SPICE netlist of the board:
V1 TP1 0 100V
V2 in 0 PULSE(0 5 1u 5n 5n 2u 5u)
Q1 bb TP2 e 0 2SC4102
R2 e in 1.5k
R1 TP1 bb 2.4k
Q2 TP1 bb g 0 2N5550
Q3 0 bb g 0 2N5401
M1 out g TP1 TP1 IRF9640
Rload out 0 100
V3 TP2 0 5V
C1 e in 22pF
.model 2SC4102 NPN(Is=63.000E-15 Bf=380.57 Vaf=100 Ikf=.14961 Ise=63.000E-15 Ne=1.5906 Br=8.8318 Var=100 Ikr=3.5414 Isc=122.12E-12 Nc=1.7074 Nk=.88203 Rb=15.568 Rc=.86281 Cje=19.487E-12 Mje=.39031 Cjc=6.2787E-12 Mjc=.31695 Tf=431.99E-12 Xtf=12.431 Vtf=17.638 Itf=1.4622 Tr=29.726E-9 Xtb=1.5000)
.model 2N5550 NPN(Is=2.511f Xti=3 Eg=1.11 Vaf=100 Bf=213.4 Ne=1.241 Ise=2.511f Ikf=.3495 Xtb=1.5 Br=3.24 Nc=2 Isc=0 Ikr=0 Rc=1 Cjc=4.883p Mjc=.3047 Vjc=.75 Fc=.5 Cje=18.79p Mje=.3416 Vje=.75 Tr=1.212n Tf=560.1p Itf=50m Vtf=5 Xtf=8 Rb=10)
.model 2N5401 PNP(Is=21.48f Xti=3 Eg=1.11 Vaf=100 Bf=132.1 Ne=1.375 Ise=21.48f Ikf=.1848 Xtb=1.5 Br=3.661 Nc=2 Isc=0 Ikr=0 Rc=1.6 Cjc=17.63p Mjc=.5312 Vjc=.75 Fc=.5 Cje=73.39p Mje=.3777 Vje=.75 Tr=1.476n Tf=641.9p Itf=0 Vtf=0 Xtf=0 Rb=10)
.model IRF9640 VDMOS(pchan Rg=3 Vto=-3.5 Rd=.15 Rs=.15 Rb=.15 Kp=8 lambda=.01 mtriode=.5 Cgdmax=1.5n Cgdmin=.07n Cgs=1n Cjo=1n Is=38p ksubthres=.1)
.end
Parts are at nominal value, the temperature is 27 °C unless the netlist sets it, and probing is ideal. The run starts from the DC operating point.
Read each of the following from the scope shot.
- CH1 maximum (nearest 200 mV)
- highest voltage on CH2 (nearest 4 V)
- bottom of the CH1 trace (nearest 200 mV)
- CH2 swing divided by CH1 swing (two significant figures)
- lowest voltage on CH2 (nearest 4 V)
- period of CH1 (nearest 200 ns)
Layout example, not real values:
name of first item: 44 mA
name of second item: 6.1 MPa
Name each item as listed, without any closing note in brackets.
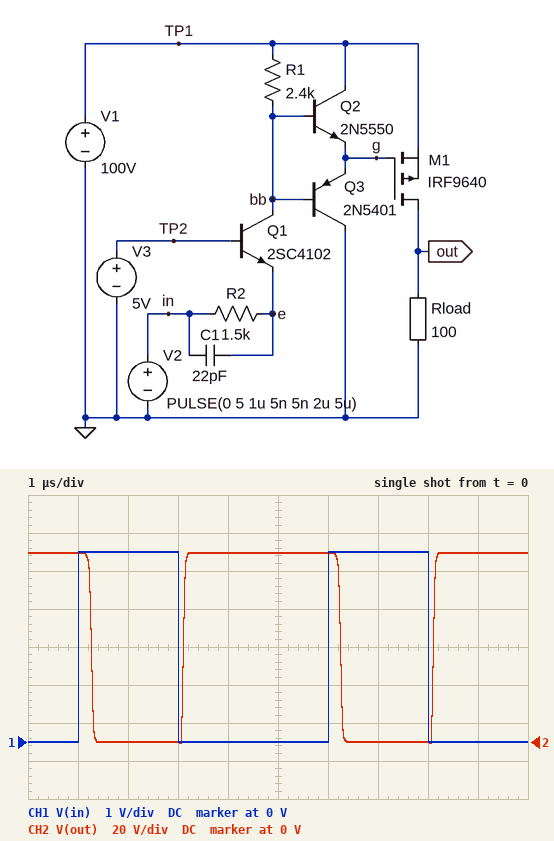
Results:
CH1 maximum: 5.0 V
highest voltage on CH2: 100 V
bottom of the CH1 trace: 0 V
CH2 swing divided by CH1 swing: 20
lowest voltage on CH2: 0 V
period of CH1: 5.0 µs
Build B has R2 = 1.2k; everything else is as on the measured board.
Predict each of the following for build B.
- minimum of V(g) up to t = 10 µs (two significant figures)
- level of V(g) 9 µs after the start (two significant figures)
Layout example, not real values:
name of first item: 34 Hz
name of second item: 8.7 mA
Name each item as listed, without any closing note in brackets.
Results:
minimum of V(g) up to t = 10 µs: 90 V
level of V(g) 9 µs after the start: 91 V
